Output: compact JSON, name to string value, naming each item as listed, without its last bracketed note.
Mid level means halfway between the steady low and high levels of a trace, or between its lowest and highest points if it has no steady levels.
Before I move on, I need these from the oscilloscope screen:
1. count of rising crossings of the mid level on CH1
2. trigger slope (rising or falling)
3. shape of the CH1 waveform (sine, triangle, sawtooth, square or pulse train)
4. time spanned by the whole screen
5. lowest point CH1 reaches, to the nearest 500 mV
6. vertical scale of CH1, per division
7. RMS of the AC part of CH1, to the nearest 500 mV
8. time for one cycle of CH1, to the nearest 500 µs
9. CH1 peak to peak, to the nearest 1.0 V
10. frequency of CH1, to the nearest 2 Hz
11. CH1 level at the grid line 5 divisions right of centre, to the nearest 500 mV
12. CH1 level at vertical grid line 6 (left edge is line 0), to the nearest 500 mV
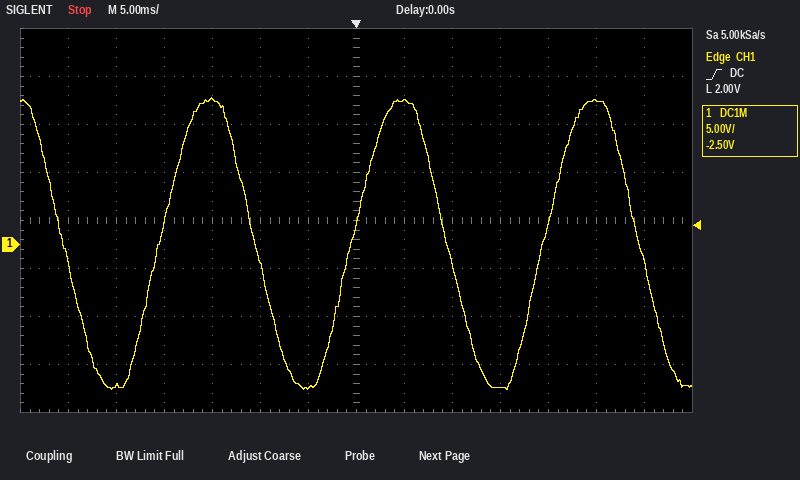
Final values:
{"count of rising crossings of the mid level on CH1": "3", "trigger slope": "rising", "shape of the CH1 waveform": "sine", "time spanned by the whole screen": "70 ms", "lowest point CH1 reaches, to the nearest 500 mV": "-15.0 V", "vertical scale of CH1, per division": "5 V", "RMS of the AC part of CH1, to the nearest 500 mV": "10.5 V", "time for one cycle of CH1, to the nearest 500 µs": "20.0 ms", "CH1 peak to peak, to the nearest 1.0 V": "30.0 V", "frequency of CH1, to the nearest 2 Hz": "50 Hz", "CH1 level at the grid line 5 divisions right of centre, to the nearest 500 mV": "15.0 V", "CH1 level at vertical grid line 6 (left edge is line 0), to the nearest 500 mV": "-15.0 V"}
